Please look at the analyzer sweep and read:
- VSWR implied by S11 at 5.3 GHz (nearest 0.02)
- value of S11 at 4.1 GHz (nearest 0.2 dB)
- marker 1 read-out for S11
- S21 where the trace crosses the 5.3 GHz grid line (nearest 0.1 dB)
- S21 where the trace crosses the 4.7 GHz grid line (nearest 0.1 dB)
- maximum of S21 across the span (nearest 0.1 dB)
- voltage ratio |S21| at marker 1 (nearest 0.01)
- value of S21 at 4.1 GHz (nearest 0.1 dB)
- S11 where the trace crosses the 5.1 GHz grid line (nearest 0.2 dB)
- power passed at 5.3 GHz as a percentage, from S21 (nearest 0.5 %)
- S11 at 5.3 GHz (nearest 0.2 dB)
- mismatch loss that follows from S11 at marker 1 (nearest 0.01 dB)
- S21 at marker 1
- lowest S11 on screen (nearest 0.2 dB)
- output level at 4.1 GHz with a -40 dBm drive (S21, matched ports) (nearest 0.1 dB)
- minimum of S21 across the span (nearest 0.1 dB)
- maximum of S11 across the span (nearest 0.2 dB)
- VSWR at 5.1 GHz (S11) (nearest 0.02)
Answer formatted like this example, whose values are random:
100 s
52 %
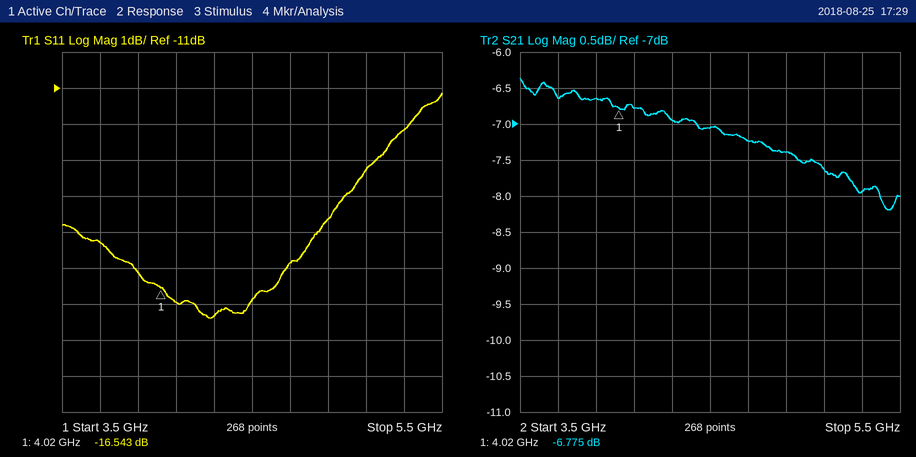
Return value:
1.66
-17.0 dB
-16.543 dB
-7.9 dB
-7.2 dB
-6.4 dB
0.46
-6.8 dB
-13.2 dB
16.0 %
-12.2 dB
0.10 dB
-6.775 dB
-17.4 dB
-46.8 dBm
-8.2 dB
-11.2 dB
1.56
